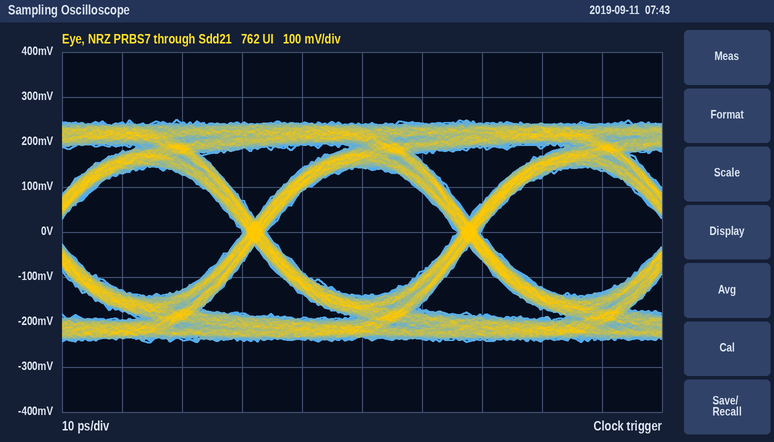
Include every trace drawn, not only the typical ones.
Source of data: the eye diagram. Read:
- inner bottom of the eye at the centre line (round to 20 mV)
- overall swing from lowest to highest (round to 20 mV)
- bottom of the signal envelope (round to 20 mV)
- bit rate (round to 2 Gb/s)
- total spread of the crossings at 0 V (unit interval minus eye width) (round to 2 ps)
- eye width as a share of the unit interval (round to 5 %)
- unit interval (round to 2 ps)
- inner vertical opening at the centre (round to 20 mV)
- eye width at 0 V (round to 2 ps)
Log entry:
-140 mV
500 mV
-240 mV
28 Gb/s
4 ps
90 %
36 ps
280 mV
32 ps
